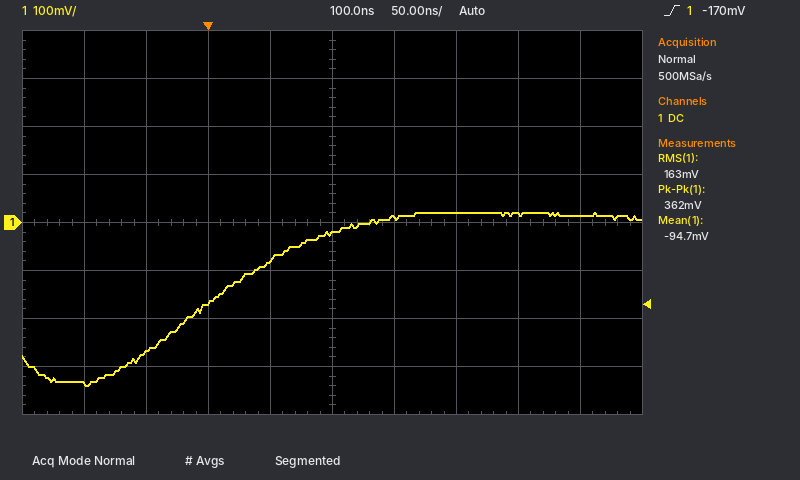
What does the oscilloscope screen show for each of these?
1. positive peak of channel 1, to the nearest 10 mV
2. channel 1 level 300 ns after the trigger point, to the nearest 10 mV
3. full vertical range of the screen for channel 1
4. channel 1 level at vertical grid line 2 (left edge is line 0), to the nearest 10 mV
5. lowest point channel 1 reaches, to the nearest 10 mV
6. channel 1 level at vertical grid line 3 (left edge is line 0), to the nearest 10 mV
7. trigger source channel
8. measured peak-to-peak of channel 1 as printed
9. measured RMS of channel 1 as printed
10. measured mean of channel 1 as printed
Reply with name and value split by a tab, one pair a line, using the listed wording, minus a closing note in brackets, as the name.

positive peak of channel 1, to the nearest 10 mV	20 mV
channel 1 level 300 ns after the trigger point, to the nearest 10 mV	10 mV
full vertical range of the screen for channel 1	800 mV
channel 1 level at vertical grid line 2 (left edge is line 0), to the nearest 10 mV	-270 mV
lowest point channel 1 reaches, to the nearest 10 mV	-340 mV
channel 1 level at vertical grid line 3 (left edge is line 0), to the nearest 10 mV	-170 mV
trigger source channel	channel 1
measured peak-to-peak of channel 1 as printed	362 mV
measured RMS of channel 1 as printed	163 mV
measured mean of channel 1 as printed	-94.7 mV
